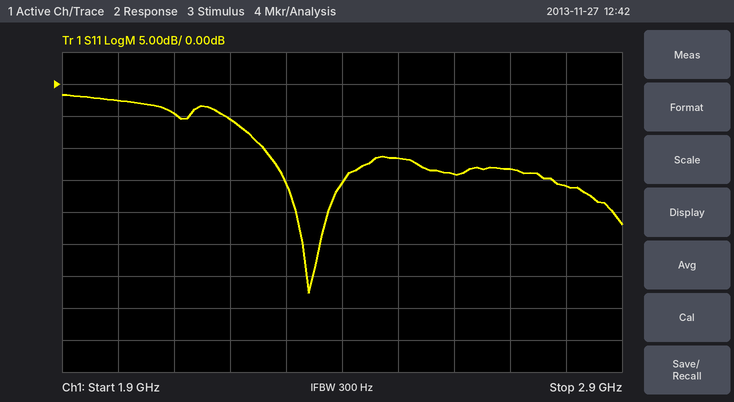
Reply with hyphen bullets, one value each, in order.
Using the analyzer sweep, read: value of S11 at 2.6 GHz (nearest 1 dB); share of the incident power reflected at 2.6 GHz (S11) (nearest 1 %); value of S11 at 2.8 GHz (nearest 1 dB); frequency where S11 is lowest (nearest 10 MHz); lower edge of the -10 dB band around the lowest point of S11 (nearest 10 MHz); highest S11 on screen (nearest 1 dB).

- -14 dB
- 4 %
- -16 dB
- 2.34 GHz
- 2.26 GHz
- -2 dB
